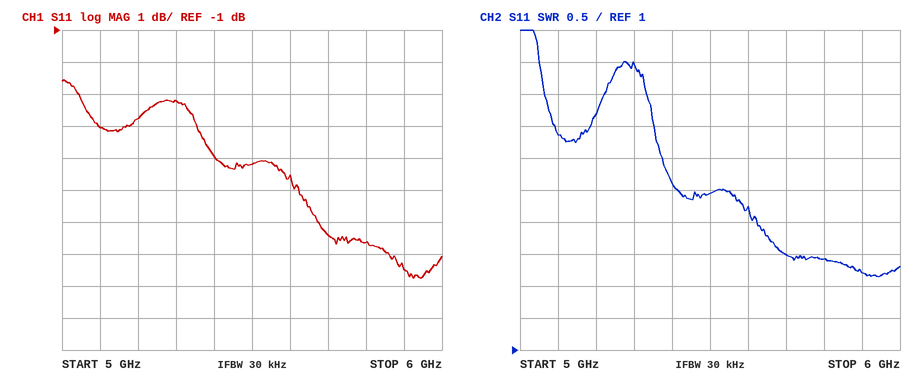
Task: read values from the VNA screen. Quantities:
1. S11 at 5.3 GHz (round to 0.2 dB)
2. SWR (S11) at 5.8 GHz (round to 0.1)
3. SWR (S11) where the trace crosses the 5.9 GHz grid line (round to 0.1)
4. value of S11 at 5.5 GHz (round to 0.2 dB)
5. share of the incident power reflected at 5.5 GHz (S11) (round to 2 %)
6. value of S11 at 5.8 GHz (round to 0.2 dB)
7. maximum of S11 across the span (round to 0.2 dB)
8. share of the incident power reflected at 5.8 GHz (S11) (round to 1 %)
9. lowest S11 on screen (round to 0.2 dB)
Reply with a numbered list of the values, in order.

1. -3.2 dB
2. 2.4
3. 2.2
4. -5.2 dB
5. 30 %
6. -7.6 dB
7. -2.6 dB
8. 17 %
9. -8.8 dB
